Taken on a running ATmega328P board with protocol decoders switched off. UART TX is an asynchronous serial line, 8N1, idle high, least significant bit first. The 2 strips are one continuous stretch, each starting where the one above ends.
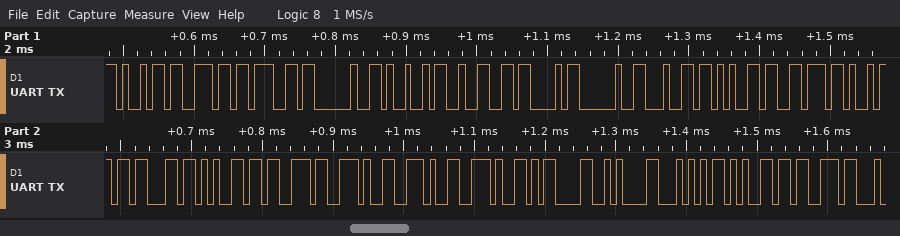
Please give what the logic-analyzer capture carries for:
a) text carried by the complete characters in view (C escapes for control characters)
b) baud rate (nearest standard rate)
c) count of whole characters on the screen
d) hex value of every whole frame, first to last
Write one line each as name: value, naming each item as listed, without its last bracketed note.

text carried by the complete characters in view: "ing I2C devices...\r\nTes"
baud rate: 115200 baud
count of whole characters on the screen: 23
hex value of every whole frame, first to last: 69 6E 67 20 49 32 43 20 64 65 76 69 63 65 73 2E 2E 2E 0D 0A 54 65 73
